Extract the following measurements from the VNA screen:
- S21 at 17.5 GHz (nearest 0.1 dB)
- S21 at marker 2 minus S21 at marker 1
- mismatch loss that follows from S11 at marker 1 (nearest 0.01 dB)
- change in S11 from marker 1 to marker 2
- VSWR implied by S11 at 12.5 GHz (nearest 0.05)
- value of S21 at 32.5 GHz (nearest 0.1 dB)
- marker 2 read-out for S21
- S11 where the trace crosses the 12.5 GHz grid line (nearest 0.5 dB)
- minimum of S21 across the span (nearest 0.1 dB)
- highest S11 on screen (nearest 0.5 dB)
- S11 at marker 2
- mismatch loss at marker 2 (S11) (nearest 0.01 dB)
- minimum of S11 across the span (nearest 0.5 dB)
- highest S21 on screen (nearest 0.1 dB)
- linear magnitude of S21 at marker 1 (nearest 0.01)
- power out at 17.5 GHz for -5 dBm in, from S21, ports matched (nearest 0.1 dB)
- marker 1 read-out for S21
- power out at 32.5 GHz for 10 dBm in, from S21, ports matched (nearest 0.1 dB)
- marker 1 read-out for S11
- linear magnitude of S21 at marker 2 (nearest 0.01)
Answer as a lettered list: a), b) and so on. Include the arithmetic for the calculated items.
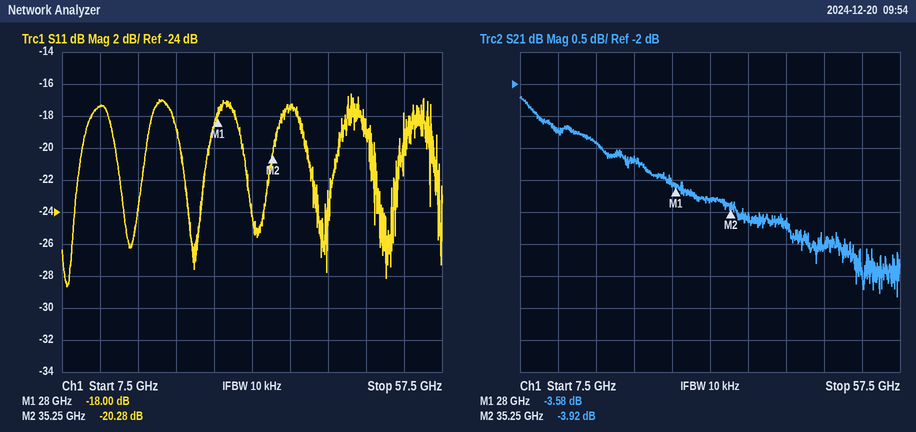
a) -2.9 dB
b) -3.92 − (-3.58) = -0.34 dB
c) −10 log10(1 − 10^(-18/10)) ≈ 0.07 dB
d) -20.28 − (-18) = -2.28 dB
e) |Γ| = 10^(-17.5/20) = 0.1334; VSWR = (1 + 0.1334)/(1 − 0.1334) ≈ 1.31, so 1.30 to the nearest 0.05
f) -3.8 dB
g) -3.92 dB
h) -17.5 dB
i) -5.3 dB
j) -16.5 dB
k) -20.28 dB
l) −10 log10(1 − 10^(-20.28/10)) ≈ 0.04 dB
m) -28.5 dB
n) -2.2 dB
o) 10^(-3.58/20) ≈ 0.66
p) -5 dBm + (-2.9 dB) = -7.9 dBm
q) -3.58 dB
r) 10 dBm + (-3.8 dB) = 6.2 dBm
s) -18.00 dB
t) 10^(-3.92/20) ≈ 0.64
